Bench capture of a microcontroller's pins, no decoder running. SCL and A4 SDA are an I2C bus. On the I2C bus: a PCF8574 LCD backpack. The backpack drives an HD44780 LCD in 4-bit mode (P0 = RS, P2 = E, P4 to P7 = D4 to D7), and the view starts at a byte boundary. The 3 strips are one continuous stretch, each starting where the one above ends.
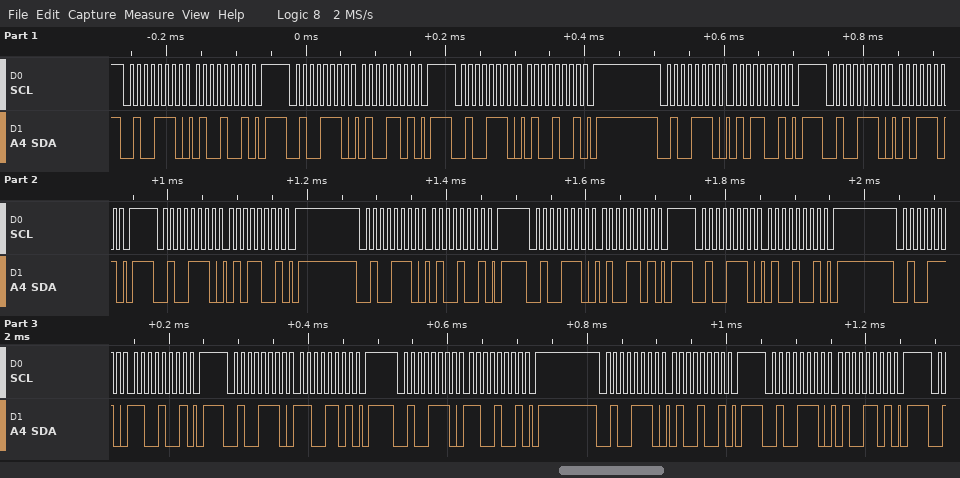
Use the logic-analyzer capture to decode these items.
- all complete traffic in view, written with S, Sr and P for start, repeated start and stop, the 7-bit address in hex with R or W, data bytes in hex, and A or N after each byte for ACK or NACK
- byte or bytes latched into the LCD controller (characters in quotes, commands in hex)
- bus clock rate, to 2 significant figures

S 27W A 49 A P S 27W A 4D A P S 27W A 49 A P S 27W A 59 A P S 27W A 5D A P S 27W A 59 A P S 27W A 49 A P S 27W A 4D A P S 27W A 49 A P S 27W A C9 A P S 27W A CD A P S 27W A C9 A P S 27W A 49 A P S 27W A 4D A P
'E' 'L'
100 kHz
